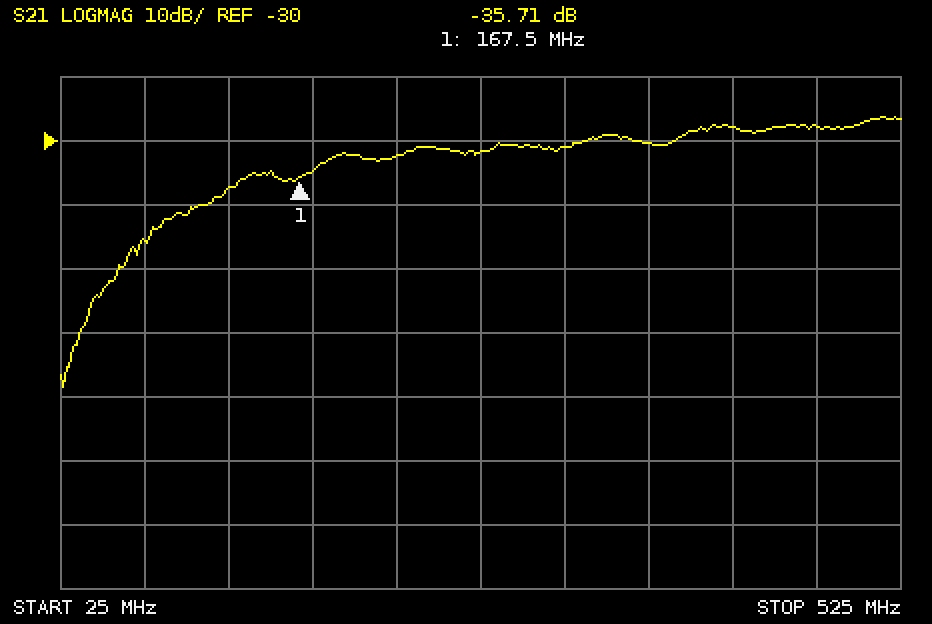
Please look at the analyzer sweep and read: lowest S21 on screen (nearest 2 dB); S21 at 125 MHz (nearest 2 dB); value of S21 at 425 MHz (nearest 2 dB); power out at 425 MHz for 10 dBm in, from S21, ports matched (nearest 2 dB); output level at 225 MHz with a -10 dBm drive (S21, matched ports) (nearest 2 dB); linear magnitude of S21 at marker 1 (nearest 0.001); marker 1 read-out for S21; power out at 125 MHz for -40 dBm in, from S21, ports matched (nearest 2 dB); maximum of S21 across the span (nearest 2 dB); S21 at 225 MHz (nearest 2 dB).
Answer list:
-68 dB
-38 dB
-28 dB
-18 dBm
-42 dBm
0.016
-35.71 dB
-78 dBm
-26 dB
-32 dB
